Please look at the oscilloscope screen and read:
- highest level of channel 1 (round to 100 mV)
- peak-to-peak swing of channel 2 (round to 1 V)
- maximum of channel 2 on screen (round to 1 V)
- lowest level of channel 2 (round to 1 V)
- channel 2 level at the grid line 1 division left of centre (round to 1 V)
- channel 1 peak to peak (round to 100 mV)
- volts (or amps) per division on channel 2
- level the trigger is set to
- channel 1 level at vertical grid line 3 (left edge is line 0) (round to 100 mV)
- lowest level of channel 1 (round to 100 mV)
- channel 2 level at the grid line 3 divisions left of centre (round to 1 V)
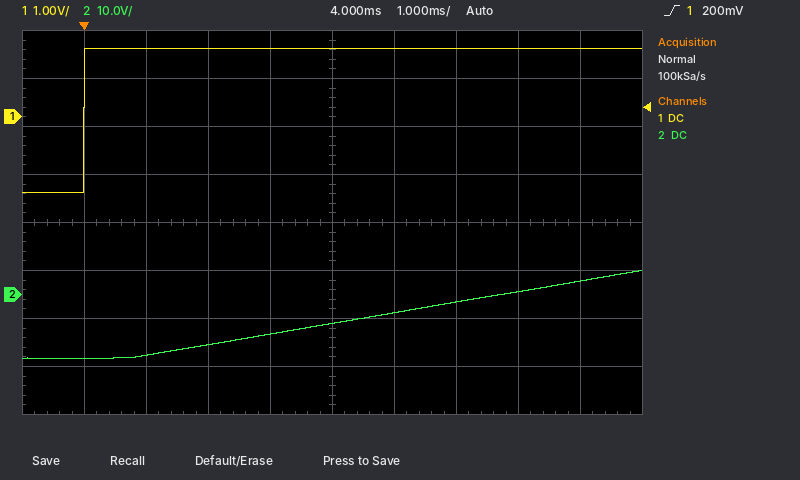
1.4 V
18 V
5 V
-13 V
-8 V
3.0 V
10 V
200 mV
1.4 V
-1.6 V
-13 V
